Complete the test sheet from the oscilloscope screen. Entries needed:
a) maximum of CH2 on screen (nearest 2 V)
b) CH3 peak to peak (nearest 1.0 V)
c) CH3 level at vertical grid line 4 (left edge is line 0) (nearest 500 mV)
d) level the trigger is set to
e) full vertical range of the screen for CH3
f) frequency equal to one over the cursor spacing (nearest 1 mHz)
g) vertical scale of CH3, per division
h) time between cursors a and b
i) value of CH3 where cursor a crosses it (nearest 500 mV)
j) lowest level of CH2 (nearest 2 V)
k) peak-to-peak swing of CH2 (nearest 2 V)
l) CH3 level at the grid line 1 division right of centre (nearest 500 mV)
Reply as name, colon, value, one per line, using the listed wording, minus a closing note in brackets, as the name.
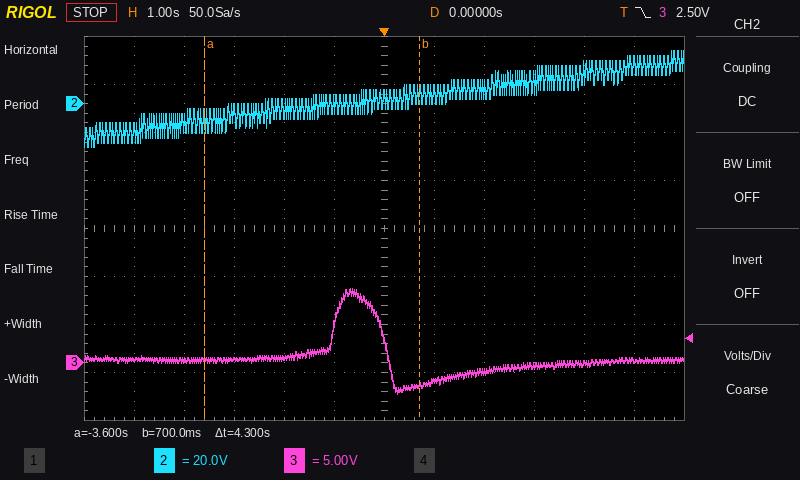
maximum of CH2 on screen: 22 V
CH3 peak to peak: 11.0 V
CH3 level at vertical grid line 4 (left edge is line 0): 500 mV
level the trigger is set to: 2.50 V
full vertical range of the screen for CH3: 40 V
frequency equal to one over the cursor spacing: 233 mHz
vertical scale of CH3, per division: 5 V
time between cursors a and b: 4.3 s
value of CH3 where cursor a crosses it: 500 mV
lowest level of CH2: -18 V
peak-to-peak swing of CH2: 40 V
CH3 level at the grid line 1 division right of centre: -2.0 V
